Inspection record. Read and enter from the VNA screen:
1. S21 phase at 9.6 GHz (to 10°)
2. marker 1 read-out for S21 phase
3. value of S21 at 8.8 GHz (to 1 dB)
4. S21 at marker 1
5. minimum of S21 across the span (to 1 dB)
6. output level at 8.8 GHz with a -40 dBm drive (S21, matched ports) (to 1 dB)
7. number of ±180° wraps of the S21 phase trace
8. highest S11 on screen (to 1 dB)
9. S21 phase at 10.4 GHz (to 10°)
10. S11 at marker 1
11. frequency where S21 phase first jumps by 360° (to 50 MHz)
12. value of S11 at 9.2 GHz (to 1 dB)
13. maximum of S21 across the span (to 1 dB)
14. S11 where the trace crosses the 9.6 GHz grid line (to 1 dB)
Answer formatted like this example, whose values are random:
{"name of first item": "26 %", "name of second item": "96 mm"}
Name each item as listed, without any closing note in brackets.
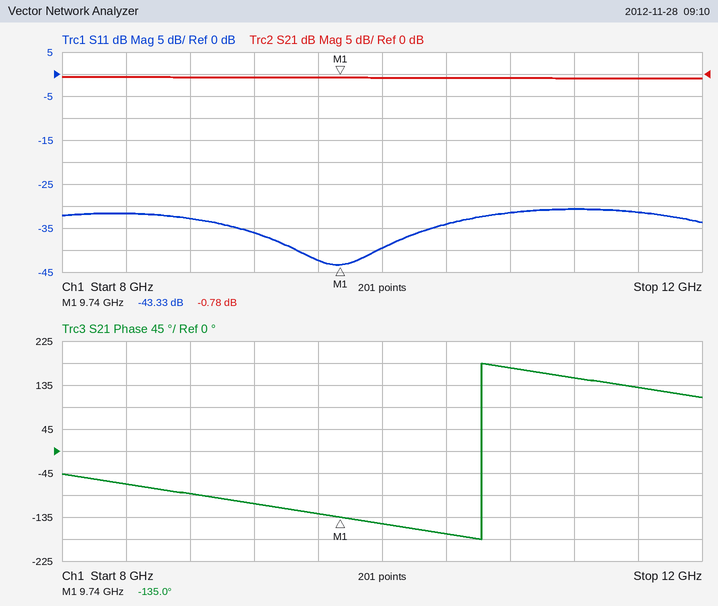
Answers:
{"S21 phase at 9.6 GHz": "-130°", "marker 1 read-out for S21 phase": "-135.0°", "value of S21 at 8.8 GHz": "-1 dB", "S21 at marker 1": "-0.78 dB", "minimum of S21 across the span": "-1 dB", "output level at 8.8 GHz with a -40 dBm drive (S21, matched ports)": "-41 dBm", "number of ±180° wraps of the S21 phase trace": "1", "highest S11 on screen": "-31 dB", "S21 phase at 10.4 GHz": "-170°", "S11 at marker 1": "-43.33 dB", "frequency where S21 phase first jumps by 360°": "10.60 GHz", "value of S11 at 9.2 GHz": "-36 dB", "maximum of S21 across the span": "-1 dB", "S11 where the trace crosses the 9.6 GHz grid line": "-42 dB"}
